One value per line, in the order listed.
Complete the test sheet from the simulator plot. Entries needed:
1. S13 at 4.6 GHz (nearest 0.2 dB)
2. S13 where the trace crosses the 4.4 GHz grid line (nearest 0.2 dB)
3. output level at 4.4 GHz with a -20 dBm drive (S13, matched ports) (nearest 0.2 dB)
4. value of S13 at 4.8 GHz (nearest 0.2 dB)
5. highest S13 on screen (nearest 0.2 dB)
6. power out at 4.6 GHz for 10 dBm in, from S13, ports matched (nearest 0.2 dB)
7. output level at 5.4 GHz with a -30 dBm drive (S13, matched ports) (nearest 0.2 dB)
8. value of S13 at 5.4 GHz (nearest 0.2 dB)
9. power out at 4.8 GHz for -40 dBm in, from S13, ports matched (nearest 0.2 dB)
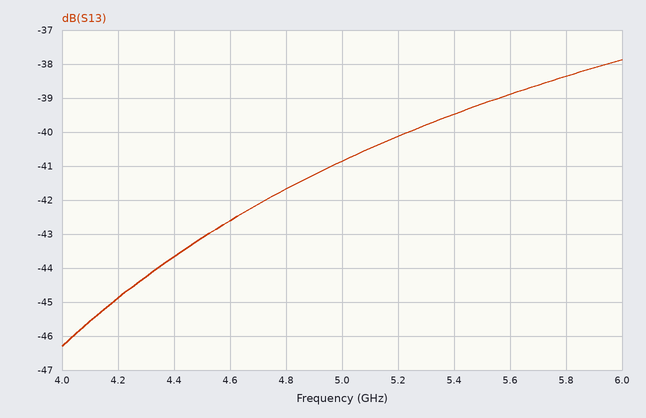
-42.6 dB
-43.6 dB
-63.6 dBm
-41.6 dB
-37.8 dB
-32.6 dBm
-69.4 dBm
-39.4 dB
-81.6 dBm
